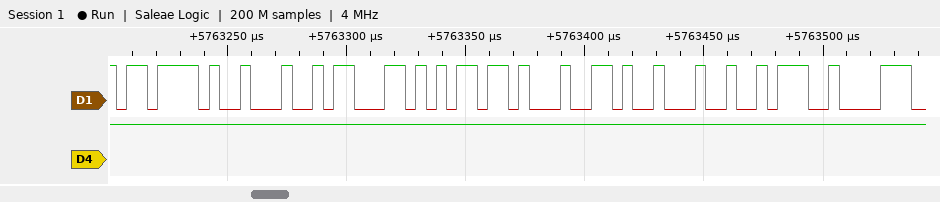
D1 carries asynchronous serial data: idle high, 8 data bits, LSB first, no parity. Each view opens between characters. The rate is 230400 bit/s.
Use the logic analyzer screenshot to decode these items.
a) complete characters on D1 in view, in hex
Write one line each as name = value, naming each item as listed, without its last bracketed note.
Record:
complete characters on D1 in view, in hex = 7B, 22, 63, 6D, 64, 22, 3A
